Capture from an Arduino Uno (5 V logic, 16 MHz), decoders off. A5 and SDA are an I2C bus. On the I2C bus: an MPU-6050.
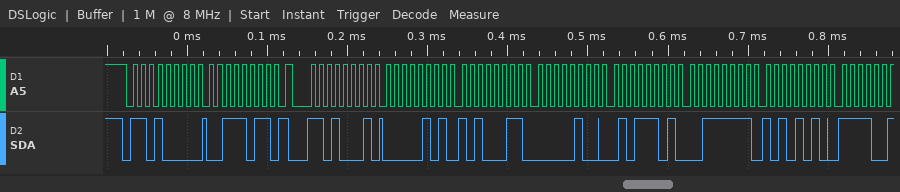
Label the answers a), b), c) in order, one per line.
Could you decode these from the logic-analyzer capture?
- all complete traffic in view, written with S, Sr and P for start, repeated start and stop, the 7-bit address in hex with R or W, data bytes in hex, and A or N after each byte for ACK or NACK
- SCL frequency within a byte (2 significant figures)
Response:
a) S 68W A 3B A Sr 68R A 05 A A3 A 04 A 5D A 3F A AA A
b) 100 kHz
